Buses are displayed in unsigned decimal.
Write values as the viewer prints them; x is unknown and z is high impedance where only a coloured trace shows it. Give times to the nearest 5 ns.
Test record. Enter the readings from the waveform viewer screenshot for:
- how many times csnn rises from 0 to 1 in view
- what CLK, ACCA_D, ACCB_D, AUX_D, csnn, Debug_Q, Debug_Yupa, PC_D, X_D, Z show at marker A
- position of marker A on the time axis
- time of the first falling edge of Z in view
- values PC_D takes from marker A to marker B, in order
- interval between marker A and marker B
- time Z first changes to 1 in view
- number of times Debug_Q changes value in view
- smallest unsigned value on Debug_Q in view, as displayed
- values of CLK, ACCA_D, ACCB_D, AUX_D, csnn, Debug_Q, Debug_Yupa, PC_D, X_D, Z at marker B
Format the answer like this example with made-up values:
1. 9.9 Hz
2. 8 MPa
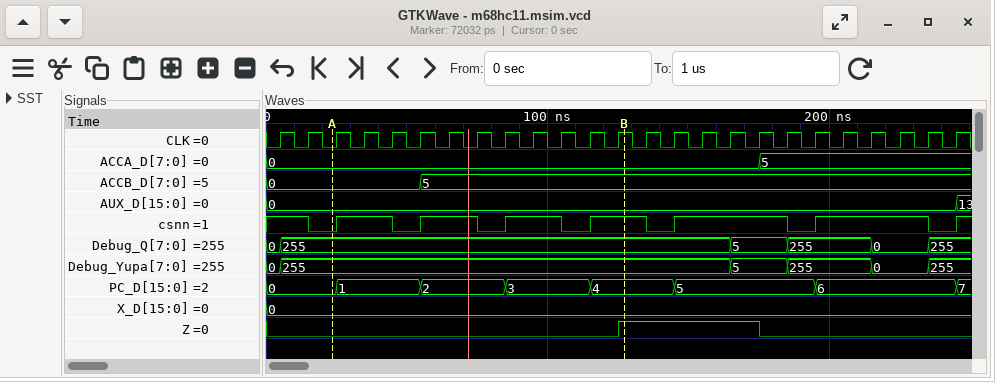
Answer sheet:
1. 7
2. CLK=0, ACCA_D=0, ACCB_D=0, AUX_D=0, csnn=0, Debug_Q=255, Debug_Yupa=255, PC_D=0, X_D=0, Z=0
3. 25 ns
4. 175 ns
5. 0, 1, 2, 3, 4
6. 105 ns
7. 125 ns
8. 5
9. 0
10. CLK=1, ACCA_D=0, ACCB_D=5, AUX_D=0, csnn=1, Debug_Q=255, Debug_Yupa=255, PC_D=4, X_D=0, Z=1
